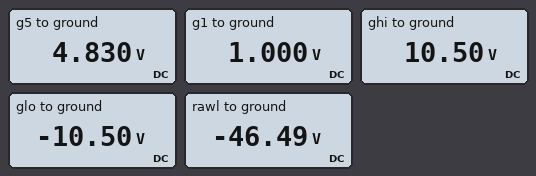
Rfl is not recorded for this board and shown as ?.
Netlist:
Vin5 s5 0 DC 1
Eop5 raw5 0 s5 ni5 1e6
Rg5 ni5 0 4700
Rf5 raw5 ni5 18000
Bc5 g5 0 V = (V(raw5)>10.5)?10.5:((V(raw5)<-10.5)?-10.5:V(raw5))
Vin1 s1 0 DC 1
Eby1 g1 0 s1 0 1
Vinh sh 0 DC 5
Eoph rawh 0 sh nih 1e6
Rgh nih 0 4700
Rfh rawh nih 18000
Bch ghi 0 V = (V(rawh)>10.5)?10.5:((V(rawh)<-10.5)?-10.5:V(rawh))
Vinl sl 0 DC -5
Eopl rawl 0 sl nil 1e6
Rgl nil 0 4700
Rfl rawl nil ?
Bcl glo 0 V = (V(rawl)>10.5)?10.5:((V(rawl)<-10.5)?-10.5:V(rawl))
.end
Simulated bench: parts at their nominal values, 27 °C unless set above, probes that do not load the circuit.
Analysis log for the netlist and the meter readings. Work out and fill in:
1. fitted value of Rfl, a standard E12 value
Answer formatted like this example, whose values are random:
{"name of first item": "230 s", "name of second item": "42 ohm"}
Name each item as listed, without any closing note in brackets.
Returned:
{"fitted value of Rfl, a standard E12 value": "39 kΩ"}
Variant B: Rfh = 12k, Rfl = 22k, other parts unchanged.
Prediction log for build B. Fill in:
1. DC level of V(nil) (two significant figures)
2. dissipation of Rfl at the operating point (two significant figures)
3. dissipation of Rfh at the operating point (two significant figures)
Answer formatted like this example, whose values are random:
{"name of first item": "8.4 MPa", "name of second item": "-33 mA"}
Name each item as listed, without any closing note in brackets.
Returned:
{"DC level of V(nil)": "-5.0 V", "dissipation of Rfl at the operating point": "25 mW", "dissipation of Rfh at the operating point": "14 mW"}
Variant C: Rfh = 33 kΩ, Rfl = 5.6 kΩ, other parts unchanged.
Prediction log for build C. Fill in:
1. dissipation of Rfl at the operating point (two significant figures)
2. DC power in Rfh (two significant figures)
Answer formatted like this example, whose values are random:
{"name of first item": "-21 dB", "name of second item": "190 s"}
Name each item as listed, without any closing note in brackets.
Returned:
{"dissipation of Rfl at the operating point": "6.3 mW", "DC power in Rfh": "37 mW"}
